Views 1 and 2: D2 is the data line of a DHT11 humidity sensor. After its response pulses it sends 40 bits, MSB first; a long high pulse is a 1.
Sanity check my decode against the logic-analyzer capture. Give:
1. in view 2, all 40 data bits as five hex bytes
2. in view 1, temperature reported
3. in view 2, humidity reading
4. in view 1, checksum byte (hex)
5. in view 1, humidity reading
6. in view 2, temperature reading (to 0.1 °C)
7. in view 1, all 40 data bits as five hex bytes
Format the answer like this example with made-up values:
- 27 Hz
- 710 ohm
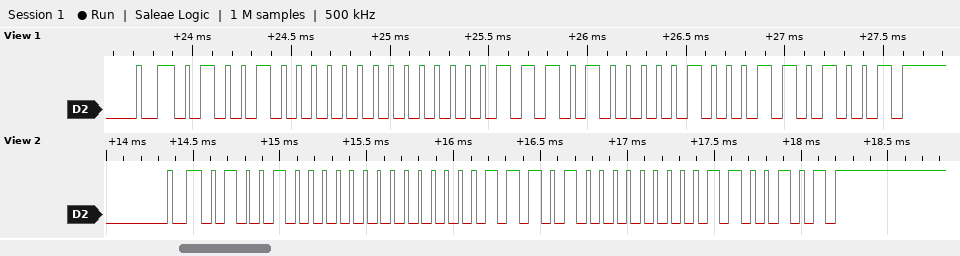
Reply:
- 48 00 1D 00 65
- 29.4 °C
- 72 %
- 0x69
- 72 %
- 29.0 °C
- 48 00 1D 04 69
